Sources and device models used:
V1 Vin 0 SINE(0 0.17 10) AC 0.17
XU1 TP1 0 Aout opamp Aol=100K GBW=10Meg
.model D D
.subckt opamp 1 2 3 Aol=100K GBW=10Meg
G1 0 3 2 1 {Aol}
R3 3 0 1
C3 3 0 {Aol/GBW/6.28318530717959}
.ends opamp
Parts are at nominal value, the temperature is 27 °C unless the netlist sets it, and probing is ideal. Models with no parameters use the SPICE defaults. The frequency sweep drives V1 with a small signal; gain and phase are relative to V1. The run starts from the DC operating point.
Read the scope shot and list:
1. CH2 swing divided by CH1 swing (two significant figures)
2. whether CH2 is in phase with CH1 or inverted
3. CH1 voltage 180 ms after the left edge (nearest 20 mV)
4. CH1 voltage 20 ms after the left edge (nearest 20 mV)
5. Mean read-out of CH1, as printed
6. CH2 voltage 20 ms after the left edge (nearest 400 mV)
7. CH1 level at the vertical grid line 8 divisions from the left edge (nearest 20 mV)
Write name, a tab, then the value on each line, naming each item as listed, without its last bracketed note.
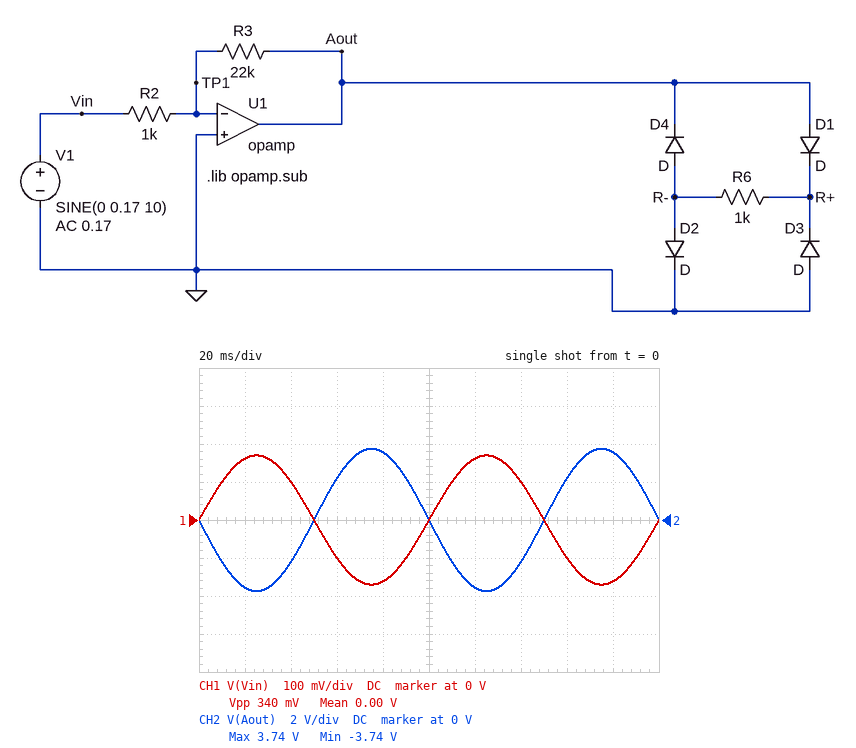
CH2 swing divided by CH1 swing	22
whether CH2 is in phase with CH1 or inverted	inverted
CH1 voltage 180 ms after the left edge	-160 mV
CH1 voltage 20 ms after the left edge	160 mV
Mean read-out of CH1, as printed	0.00 V
CH2 voltage 20 ms after the left edge	-3.6 V
CH1 level at the vertical grid line 8 divisions from the left edge	-100 mV
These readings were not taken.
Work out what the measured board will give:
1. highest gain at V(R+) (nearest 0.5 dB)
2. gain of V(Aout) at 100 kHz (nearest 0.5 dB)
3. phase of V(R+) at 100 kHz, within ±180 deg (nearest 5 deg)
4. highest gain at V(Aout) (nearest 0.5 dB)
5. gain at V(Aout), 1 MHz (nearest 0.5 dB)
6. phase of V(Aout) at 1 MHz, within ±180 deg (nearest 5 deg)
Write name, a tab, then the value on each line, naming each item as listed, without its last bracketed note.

highest gain at V(R+)	21.0 dB
gain of V(Aout) at 100 kHz	26.5 dB
phase of V(R+) at 100 kHz, within ±180 deg	165 deg
highest gain at V(Aout)	27.0 dB
gain at V(Aout), 1 MHz	19.0 dB
phase of V(Aout) at 1 MHz, within ±180 deg	115 deg
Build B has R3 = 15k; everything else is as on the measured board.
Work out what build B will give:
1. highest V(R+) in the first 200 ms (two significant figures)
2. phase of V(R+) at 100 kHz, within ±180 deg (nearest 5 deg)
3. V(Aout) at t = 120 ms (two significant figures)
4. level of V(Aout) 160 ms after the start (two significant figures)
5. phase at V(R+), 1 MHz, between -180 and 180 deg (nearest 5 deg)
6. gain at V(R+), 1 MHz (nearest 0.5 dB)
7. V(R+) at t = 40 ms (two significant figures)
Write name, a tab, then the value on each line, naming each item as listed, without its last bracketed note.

highest V(R+) in the first 200 ms	1.9 V
phase of V(R+) at 100 kHz, within ±180 deg	170 deg
V(Aout) at t = 120 ms	-2.4 V
level of V(Aout) 160 ms after the start	1.5 V
phase at V(R+), 1 MHz, between -180 and 180 deg	120 deg
gain at V(R+), 1 MHz	12.0 dB
V(R+) at t = 40 ms	-620 mV
